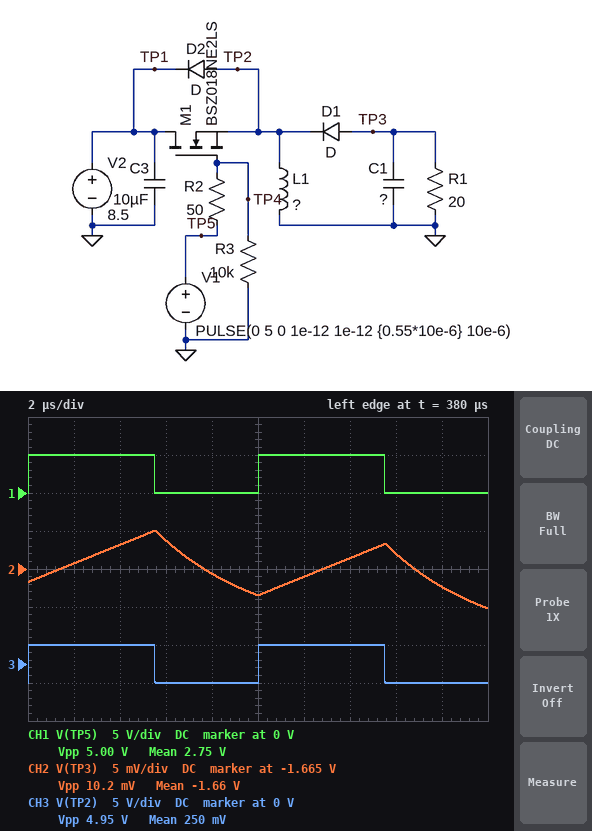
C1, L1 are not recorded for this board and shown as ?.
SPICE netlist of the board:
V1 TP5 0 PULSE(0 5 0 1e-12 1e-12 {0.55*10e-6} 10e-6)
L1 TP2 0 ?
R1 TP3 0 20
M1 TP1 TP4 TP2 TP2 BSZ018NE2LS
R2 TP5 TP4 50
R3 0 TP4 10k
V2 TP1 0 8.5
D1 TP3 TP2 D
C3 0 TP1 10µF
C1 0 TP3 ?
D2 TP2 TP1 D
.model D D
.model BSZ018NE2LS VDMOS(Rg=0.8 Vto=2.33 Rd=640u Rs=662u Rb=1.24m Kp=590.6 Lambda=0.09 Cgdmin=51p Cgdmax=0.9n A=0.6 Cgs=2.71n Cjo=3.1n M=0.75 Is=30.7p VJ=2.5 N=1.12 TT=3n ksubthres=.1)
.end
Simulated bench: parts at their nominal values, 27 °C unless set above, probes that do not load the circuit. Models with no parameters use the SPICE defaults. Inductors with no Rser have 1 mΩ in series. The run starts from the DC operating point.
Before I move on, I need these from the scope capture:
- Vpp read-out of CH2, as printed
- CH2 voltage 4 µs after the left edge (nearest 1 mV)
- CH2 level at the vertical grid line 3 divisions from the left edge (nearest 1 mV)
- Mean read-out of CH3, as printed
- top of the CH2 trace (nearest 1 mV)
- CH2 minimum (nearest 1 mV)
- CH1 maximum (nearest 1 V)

10.2 mV
-1.662 V
-1.661 V
250 mV
-1.660 V
-1.670 V
5 V
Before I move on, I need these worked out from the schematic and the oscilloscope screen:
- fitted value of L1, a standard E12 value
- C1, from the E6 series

12 µH
68 µF
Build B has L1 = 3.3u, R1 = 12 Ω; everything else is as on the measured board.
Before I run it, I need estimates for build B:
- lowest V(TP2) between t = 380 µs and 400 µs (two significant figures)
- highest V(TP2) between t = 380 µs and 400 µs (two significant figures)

-2.6 V
2.4 V
